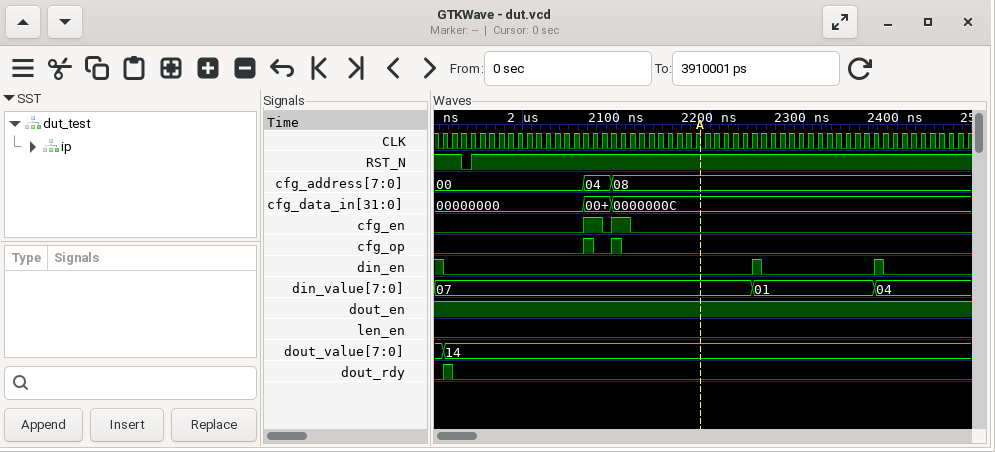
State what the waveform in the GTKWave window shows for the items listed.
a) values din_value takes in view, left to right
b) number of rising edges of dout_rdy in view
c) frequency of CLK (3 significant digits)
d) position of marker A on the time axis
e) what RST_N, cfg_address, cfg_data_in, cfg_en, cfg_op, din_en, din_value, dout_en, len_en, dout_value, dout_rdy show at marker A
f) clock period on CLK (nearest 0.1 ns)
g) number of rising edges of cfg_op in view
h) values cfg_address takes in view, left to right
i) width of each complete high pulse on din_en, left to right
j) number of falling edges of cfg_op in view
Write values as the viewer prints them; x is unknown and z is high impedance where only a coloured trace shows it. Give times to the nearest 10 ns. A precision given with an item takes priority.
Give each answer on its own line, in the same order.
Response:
07, 01, 04
1
100 MHz
2190 ns
RST_N=1, cfg_address=08, cfg_data_in=0000000C, cfg_en=0, cfg_op=0, din_en=0, din_value=07, dout_en=1, len_en=0, dout_value=14, dout_rdy=0
10 ns
2
00, 04, 08
10 ns, 10 ns
2
